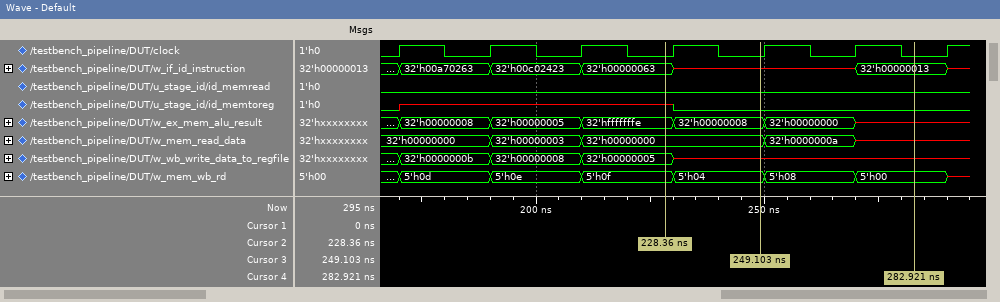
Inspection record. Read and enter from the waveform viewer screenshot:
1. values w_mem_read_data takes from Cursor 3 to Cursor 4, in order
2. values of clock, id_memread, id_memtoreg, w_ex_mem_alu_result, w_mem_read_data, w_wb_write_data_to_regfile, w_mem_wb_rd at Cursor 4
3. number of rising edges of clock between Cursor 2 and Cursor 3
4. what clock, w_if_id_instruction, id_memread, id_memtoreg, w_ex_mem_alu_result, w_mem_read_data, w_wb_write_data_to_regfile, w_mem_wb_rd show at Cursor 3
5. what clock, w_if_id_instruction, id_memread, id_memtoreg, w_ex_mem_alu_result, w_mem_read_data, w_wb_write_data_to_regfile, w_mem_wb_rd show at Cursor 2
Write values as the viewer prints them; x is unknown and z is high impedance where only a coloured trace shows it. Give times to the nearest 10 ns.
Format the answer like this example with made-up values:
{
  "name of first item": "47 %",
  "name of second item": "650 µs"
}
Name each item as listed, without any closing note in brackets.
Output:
{
  "values w_mem_read_data takes from Cursor 3 to Cursor 4, in order": "32'h00000000, 32'h0000000a, x",
  "values of clock, id_memread, id_memtoreg, w_ex_mem_alu_result, w_mem_read_data, w_wb_write_data_to_regfile, w_mem_wb_rd at Cursor 4": "clock=0, id_memread=0, id_memtoreg=0, w_ex_mem_alu_result=x, w_mem_read_data=x, w_wb_write_data_to_regfile=x, w_mem_wb_rd=5'h00",
  "number of rising edges of clock between Cursor 2 and Cursor 3": "1",
  "what clock, w_if_id_instruction, id_memread, id_memtoreg, w_ex_mem_alu_result, w_mem_read_data, w_wb_write_data_to_regfile, w_mem_wb_rd show at Cursor 3": "clock=0, w_if_id_instruction=x, id_memread=0, id_memtoreg=0, w_ex_mem_alu_result=32'h00000008, w_mem_read_data=32'h00000000, w_wb_write_data_to_regfile=x, w_mem_wb_rd=5'h04",
  "what clock, w_if_id_instruction, id_memread, id_memtoreg, w_ex_mem_alu_result, w_mem_read_data, w_wb_write_data_to_regfile, w_mem_wb_rd show at Cursor 2": "clock=0, w_if_id_instruction=32'h00000063, id_memread=0, id_memtoreg=x, w_ex_mem_alu_result=32'hfffffffe, w_mem_read_data=32'h00000000, w_wb_write_data_to_regfile=32'h00000005, w_mem_wb_rd=5'h0f"
}
